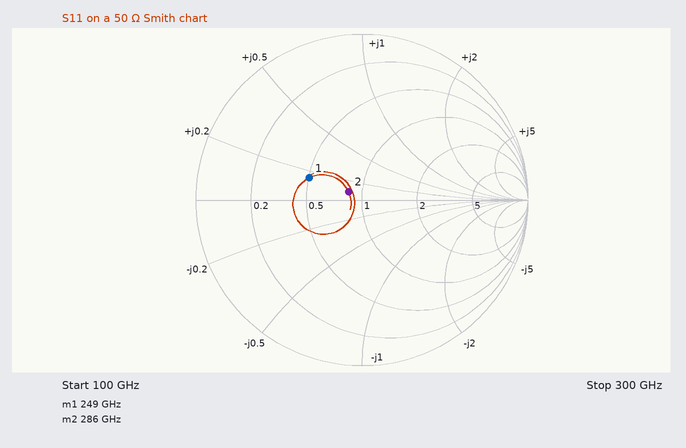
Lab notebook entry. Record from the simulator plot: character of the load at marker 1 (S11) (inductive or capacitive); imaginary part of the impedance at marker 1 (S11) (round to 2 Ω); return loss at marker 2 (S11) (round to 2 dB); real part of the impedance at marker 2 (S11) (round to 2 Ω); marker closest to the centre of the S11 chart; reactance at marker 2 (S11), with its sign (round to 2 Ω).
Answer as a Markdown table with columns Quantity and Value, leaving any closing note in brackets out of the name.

| Quantity | Value |
|---|---|
| character of the load at marker 1 (S11) | inductive |
| imaginary part of the impedance at marker 1 (S11) | +8 Ω |
| return loss at marker 2 (S11) | 20 dB |
| real part of the impedance at marker 2 (S11) | 42 Ω |
| marker closest to the centre of the S11 chart | marker 2 |
| reactance at marker 2 (S11), with its sign | +4 Ω |
